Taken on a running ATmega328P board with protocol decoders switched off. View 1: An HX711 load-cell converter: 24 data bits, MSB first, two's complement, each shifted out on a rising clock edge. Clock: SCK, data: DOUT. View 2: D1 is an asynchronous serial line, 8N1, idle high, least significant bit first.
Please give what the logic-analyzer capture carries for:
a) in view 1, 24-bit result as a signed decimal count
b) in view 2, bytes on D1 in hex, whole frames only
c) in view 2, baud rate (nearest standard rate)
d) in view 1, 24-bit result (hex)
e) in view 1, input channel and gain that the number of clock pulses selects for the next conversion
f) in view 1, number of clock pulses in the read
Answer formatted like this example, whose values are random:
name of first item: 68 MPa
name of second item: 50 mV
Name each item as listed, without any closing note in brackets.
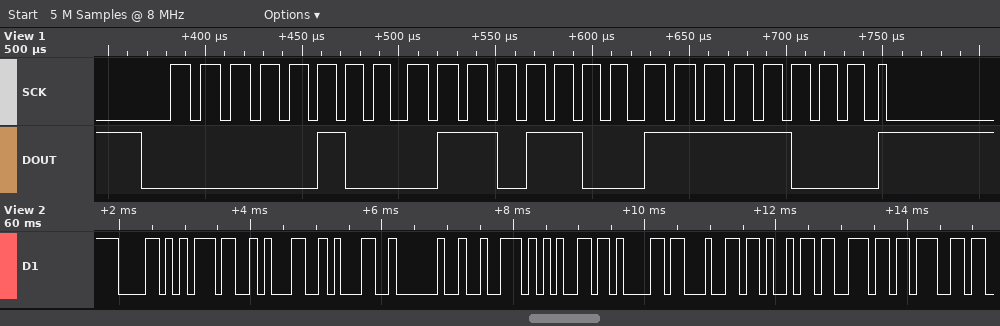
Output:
in view 1, 24-bit result as a signed decimal count: 290040
in view 2, bytes on D1 in hex, whole frames only: 58 37 31 31 20 72 65 61 64 69 6E 67
in view 2, baud rate: 9600 baud
in view 1, 24-bit result: 0x046CF8
in view 1, input channel and gain that the number of clock pulses selects for the next conversion: channel A, gain 128
in view 1, number of clock pulses in the read: 25
